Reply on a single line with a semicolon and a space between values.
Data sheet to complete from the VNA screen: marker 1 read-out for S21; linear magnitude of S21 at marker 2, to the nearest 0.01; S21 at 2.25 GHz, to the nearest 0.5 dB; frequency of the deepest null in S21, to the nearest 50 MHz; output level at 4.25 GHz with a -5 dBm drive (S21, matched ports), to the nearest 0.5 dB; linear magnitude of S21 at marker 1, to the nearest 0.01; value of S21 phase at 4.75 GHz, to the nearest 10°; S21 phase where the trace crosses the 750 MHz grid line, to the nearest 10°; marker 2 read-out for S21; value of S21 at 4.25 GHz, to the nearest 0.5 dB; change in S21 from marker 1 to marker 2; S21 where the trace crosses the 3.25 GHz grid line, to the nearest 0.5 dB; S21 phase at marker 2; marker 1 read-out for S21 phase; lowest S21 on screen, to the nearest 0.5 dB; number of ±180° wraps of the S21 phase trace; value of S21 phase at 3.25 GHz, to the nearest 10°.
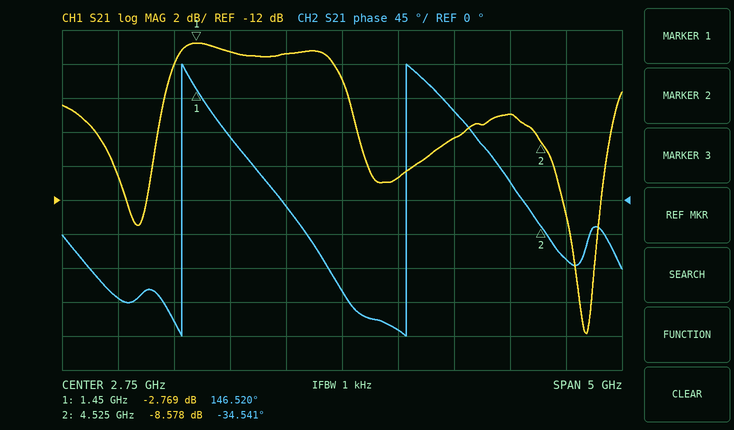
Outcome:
-2.769 dB; 0.37; -3.5 dB; 4.95 GHz; -12.0 dBm; 0.73; -80°; -130°; -8.578 dB; -7.0 dB; -5.809 dB; -10.5 dB; -34.541°; 146.520°; -20.0 dB; 2; -170°
